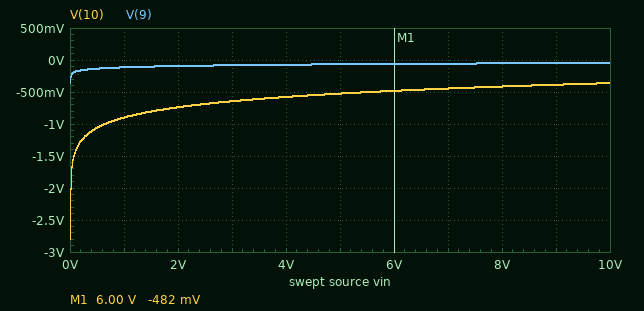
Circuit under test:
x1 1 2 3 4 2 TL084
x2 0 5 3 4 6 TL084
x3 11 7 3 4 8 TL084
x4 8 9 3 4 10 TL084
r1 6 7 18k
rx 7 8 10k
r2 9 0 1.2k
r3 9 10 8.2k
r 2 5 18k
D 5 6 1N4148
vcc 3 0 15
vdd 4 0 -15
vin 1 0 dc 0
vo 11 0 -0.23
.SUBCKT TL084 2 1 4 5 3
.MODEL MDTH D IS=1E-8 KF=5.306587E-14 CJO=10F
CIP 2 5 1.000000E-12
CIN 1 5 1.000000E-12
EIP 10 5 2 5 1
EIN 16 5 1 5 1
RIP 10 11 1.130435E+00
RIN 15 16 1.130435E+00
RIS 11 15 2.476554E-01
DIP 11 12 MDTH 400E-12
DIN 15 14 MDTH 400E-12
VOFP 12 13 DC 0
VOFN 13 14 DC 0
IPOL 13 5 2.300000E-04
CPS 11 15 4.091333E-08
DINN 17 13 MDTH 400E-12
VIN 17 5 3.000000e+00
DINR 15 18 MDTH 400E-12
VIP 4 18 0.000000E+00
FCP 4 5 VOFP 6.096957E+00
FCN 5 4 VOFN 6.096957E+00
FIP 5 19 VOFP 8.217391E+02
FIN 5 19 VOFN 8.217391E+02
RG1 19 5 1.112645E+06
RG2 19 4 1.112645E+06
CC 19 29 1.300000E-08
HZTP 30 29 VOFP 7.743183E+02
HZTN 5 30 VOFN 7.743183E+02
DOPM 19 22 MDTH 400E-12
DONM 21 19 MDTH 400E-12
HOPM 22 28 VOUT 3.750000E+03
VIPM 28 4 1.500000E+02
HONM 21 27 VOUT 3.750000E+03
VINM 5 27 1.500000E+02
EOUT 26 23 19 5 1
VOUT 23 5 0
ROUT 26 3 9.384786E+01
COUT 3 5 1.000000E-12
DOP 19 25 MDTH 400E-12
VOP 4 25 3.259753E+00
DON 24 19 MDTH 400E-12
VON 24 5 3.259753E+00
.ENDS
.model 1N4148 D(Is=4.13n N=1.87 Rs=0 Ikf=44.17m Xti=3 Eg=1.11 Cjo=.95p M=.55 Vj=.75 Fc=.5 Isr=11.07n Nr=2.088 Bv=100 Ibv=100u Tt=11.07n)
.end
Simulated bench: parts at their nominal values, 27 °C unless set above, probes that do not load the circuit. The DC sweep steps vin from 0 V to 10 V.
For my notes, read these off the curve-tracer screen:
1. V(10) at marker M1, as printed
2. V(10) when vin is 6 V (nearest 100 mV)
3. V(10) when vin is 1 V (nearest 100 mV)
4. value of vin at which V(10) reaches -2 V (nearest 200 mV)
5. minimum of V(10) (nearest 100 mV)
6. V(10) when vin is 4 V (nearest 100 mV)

-482 mV
-500 mV
-900 mV
0 V
-2.8 V
-600 mV
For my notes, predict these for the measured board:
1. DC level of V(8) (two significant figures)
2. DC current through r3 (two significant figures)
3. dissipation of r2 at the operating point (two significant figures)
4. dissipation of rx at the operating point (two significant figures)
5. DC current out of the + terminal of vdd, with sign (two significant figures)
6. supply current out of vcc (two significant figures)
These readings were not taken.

-360 mV
300 µA
110 µW
1.6 µW
-6.0 mA
5.7 mA
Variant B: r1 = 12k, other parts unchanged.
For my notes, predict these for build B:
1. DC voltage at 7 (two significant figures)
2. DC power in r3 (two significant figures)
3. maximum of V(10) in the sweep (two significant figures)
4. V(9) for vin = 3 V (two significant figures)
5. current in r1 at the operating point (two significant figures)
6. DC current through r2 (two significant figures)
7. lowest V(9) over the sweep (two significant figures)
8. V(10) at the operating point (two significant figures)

-230 mV
1.0 mW
360 mV
-8.4 mV
19 µA
350 µA
-420 mV
-3.3 V
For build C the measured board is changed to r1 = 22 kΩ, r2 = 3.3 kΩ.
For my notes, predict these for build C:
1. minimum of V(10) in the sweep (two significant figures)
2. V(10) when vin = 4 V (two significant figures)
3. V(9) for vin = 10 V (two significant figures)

-1.2 V
-360 mV
-80 mV
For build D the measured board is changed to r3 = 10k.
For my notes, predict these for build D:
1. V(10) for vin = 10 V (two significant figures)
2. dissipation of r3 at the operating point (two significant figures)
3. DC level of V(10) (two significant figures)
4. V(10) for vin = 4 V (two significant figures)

-430 mV
890 µW
-3.3 V
-690 mV
